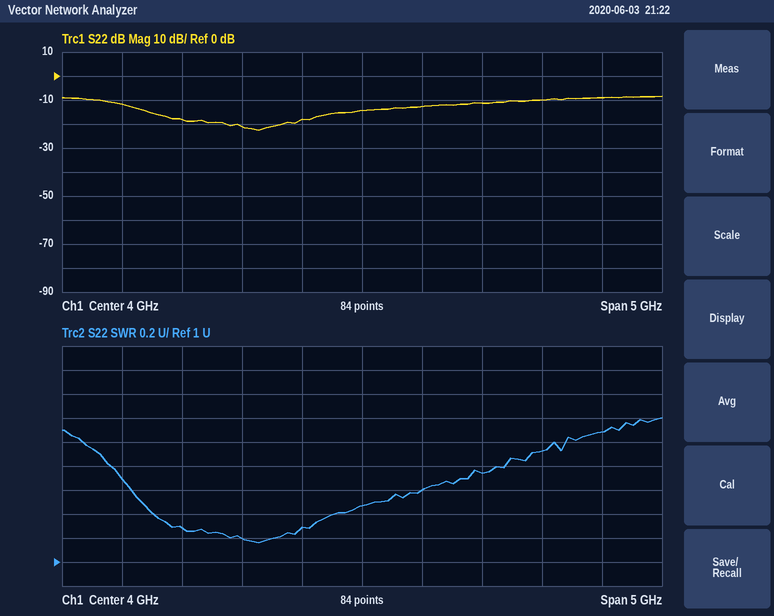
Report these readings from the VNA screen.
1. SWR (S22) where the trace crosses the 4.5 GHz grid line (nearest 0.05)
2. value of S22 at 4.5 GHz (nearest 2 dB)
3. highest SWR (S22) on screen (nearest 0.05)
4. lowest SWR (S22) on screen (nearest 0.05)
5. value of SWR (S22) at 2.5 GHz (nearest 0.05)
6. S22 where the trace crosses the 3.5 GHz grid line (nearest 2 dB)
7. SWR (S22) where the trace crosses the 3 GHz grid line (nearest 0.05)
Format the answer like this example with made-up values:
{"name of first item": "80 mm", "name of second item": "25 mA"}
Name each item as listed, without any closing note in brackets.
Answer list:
{"SWR (S22) where the trace crosses the 4.5 GHz grid line": "1.60", "value of S22 at 4.5 GHz": "-12 dB", "highest SWR (S22) on screen": "2.20", "lowest SWR (S22) on screen": "1.15", "value of SWR (S22) at 2.5 GHz": "1.30", "S22 where the trace crosses the 3.5 GHz grid line": "-18 dB", "SWR (S22) where the trace crosses the 3 GHz grid line": "1.20"}
